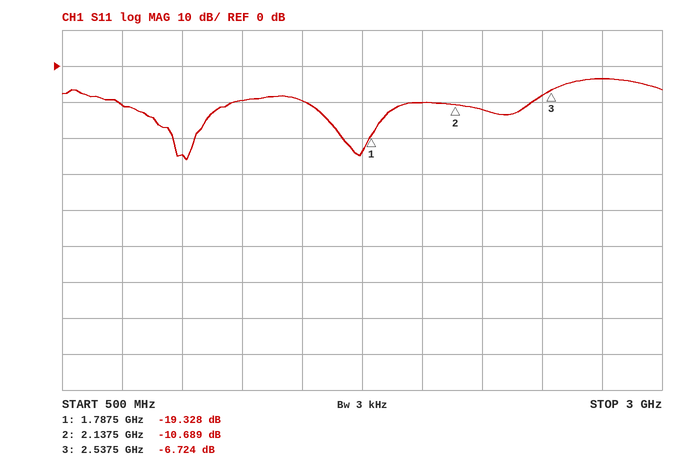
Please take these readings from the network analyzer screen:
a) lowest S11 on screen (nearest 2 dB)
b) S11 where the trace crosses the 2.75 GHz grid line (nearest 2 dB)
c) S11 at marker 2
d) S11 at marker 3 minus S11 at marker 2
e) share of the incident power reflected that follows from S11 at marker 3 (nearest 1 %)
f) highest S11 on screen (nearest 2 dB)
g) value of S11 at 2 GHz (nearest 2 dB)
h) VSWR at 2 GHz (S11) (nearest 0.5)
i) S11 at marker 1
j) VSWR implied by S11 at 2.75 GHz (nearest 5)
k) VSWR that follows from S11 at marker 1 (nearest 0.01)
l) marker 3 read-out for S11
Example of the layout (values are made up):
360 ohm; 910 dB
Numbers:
-26 dB; -4 dB; -10.689 dB; 3.965 dB; 21 %; -4 dB; -10 dB; 2.0; -19.328 dB; 5; 1.24; -6.724 dB
